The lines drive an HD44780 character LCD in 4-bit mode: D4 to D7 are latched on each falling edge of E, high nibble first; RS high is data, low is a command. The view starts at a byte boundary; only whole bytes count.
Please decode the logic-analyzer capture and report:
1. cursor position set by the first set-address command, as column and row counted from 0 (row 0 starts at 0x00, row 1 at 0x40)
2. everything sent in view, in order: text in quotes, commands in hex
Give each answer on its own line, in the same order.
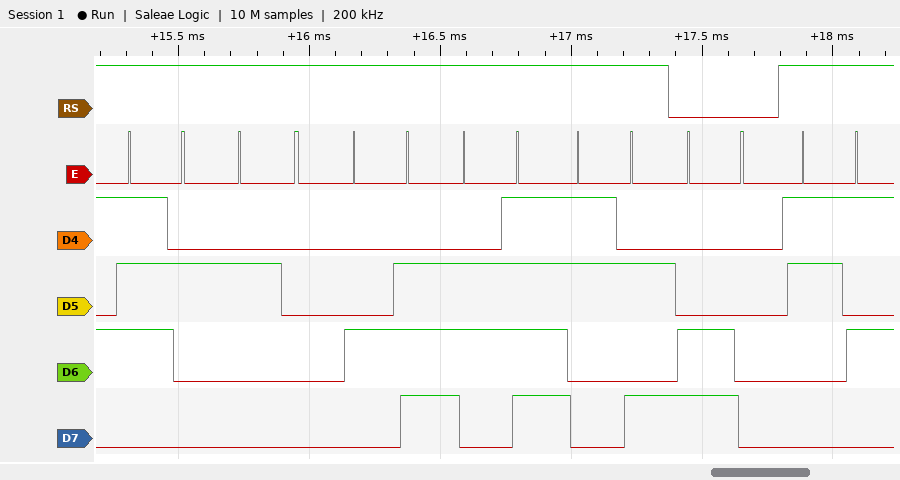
column 0, row 1
"r No:" 0xC0 "5"
